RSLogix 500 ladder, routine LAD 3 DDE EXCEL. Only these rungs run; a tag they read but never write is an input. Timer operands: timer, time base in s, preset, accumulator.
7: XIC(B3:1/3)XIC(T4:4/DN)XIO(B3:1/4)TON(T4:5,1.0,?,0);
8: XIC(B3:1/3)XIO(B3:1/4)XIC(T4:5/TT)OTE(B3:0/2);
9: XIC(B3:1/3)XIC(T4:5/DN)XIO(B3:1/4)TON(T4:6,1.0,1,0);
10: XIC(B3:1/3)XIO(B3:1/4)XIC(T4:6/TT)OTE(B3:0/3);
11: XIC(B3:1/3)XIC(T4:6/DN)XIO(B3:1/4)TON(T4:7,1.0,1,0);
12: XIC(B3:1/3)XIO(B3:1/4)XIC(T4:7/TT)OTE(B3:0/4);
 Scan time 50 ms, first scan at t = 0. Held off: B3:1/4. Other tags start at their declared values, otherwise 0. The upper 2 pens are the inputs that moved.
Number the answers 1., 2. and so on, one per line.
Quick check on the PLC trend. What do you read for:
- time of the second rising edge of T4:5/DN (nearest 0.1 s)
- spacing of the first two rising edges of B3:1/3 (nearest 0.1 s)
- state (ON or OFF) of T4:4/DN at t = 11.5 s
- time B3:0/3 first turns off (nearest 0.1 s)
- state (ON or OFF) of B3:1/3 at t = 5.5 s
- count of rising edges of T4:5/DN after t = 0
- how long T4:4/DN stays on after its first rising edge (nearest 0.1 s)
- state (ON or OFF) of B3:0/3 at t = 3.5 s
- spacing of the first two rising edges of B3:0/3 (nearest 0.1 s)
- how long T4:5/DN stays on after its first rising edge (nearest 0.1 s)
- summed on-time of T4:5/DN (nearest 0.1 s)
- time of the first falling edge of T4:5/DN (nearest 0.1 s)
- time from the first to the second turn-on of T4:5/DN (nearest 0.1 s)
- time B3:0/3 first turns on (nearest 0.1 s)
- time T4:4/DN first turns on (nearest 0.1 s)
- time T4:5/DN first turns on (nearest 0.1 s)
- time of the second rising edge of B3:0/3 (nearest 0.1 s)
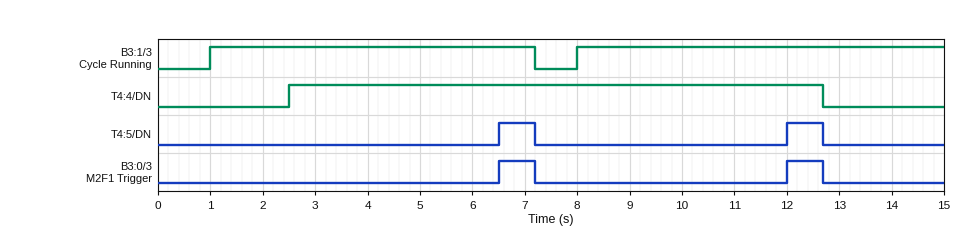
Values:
1. 12.0 s
2. 7.0 s
3. ON
4. 7.2 s
5. ON
6. 2
7. 10.2 s
8. OFF
9. 5.5 s
10. 0.7 s
11. 1.4 s
12. 7.2 s
13. 5.5 s
14. 6.5 s
15. 2.5 s
16. 6.5 s
17. 12.0 s
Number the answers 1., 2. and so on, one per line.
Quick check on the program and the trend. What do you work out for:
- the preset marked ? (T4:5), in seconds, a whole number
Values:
1. 4 s
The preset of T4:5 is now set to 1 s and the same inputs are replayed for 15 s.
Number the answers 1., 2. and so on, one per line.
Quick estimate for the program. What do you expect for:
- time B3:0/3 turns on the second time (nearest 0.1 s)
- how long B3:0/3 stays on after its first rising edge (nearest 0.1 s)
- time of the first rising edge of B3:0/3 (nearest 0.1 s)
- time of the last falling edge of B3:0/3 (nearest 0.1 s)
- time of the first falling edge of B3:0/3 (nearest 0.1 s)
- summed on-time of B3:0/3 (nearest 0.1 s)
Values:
1. 9.0 s
2. 1.0 s
3. 3.5 s
4. 10.0 s
5. 4.5 s
6. 2.0 s
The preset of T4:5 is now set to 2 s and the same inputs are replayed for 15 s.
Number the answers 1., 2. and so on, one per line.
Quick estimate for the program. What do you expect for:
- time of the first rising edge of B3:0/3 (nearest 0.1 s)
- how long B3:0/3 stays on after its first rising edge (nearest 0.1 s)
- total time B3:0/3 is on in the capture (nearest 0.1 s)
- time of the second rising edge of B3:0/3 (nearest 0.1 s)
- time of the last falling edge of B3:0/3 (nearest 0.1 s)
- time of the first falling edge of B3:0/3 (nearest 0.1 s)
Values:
1. 4.5 s
2. 1.0 s
3. 2.0 s
4. 10.0 s
5. 11.0 s
6. 5.5 s
